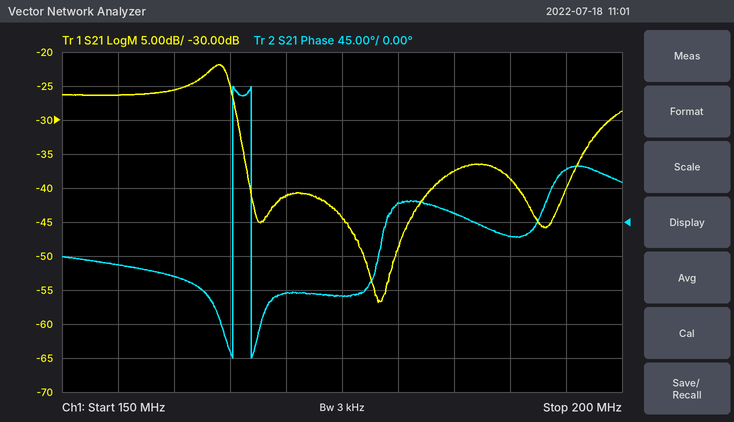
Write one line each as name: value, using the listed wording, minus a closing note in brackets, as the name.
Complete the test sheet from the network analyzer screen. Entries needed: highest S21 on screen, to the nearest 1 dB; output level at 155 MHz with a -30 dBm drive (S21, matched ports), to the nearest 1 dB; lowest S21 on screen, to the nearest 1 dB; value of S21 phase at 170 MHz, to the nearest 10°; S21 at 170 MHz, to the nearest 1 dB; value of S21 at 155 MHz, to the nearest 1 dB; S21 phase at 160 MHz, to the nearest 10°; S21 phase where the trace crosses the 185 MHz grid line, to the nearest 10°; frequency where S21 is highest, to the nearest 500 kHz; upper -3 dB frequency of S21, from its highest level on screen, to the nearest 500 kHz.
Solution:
highest S21 on screen, to the nearest 1 dB: -22 dB
output level at 155 MHz with a -30 dBm drive (S21, matched ports), to the nearest 1 dB: -56 dBm
lowest S21 on screen, to the nearest 1 dB: -57 dB
value of S21 phase at 170 MHz, to the nearest 10°: -90°
S21 at 170 MHz, to the nearest 1 dB: -41 dB
value of S21 at 155 MHz, to the nearest 1 dB: -26 dB
S21 phase at 160 MHz, to the nearest 10°: -70°
S21 phase where the trace crosses the 185 MHz grid line, to the nearest 10°: 10°
frequency where S21 is highest, to the nearest 500 kHz: 164.0 MHz
upper -3 dB frequency of S21, from its highest level on screen, to the nearest 500 kHz: 165.0 MHz
